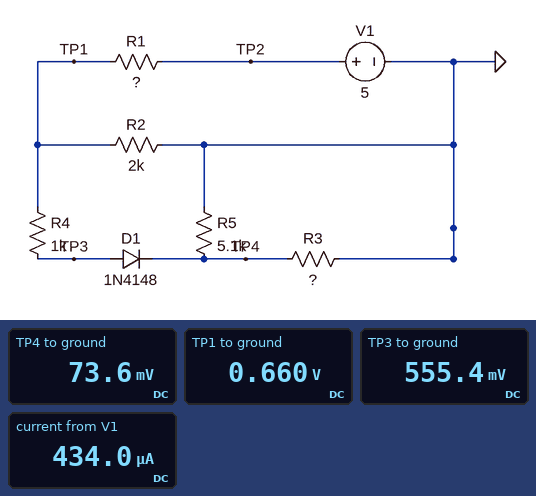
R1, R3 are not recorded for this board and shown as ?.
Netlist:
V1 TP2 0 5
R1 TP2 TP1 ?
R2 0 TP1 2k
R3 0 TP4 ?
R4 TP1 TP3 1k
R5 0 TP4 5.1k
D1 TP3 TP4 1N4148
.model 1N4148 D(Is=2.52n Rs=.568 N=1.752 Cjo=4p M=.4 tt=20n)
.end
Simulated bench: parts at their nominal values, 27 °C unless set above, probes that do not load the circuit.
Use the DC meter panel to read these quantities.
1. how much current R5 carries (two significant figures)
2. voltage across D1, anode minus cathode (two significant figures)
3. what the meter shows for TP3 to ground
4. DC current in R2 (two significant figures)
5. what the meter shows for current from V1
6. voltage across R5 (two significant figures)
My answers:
14 µA
480 mV
555.4 mV
330 µA
434.0 µA
74 mV
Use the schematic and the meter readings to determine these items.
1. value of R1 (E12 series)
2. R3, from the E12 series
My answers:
10 kΩ
820 Ω
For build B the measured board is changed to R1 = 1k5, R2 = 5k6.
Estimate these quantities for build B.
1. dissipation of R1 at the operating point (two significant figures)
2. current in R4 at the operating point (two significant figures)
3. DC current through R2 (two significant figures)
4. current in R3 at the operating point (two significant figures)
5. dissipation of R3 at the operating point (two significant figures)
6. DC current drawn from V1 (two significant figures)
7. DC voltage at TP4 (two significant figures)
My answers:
3.9 mW
1.2 mA
460 µA
1.0 mA
820 µW
1.6 mA
820 mV
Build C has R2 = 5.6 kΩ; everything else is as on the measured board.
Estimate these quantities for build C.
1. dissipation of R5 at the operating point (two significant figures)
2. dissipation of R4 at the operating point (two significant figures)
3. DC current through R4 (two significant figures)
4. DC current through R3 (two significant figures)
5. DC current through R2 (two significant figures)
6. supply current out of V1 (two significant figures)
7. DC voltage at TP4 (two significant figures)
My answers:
5.7 µW
58 µW
240 µA
210 µA
170 µA
410 µA
170 mV
